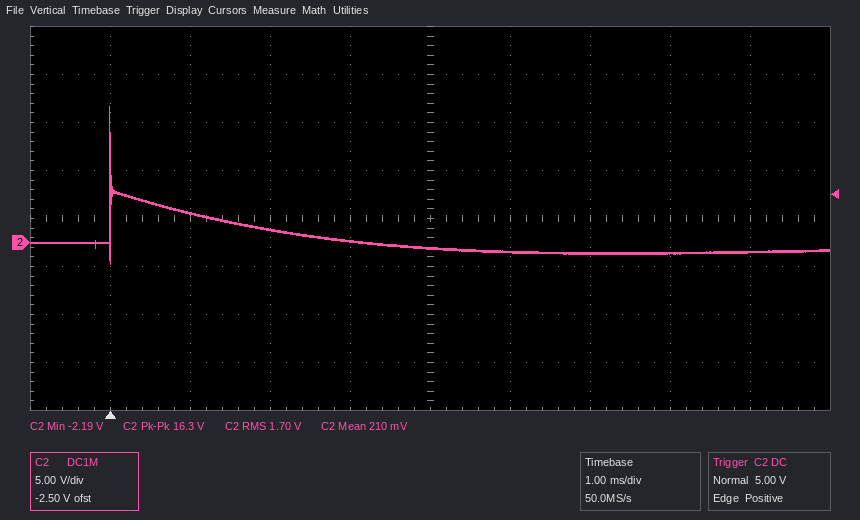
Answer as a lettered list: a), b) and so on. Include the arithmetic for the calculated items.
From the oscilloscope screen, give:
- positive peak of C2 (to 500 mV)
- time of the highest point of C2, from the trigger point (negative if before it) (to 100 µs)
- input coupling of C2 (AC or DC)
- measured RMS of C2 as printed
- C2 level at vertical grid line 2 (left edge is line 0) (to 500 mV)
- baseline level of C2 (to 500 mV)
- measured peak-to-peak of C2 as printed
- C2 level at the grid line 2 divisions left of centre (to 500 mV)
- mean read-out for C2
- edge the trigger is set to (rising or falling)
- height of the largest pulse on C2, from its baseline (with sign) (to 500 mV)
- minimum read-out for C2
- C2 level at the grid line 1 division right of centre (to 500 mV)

a) 14.0 V
b) 0.0 ms
c) DC
d) 1.70 V
e) 3.0 V
f) -1.0 V
g) 16.3 V
h) 1.5 V
i) 210 mV
j) rising
k) 14.0 V − (-1.0 V) = +15.0 V
l) -2.19 V
m) -1.0 V
